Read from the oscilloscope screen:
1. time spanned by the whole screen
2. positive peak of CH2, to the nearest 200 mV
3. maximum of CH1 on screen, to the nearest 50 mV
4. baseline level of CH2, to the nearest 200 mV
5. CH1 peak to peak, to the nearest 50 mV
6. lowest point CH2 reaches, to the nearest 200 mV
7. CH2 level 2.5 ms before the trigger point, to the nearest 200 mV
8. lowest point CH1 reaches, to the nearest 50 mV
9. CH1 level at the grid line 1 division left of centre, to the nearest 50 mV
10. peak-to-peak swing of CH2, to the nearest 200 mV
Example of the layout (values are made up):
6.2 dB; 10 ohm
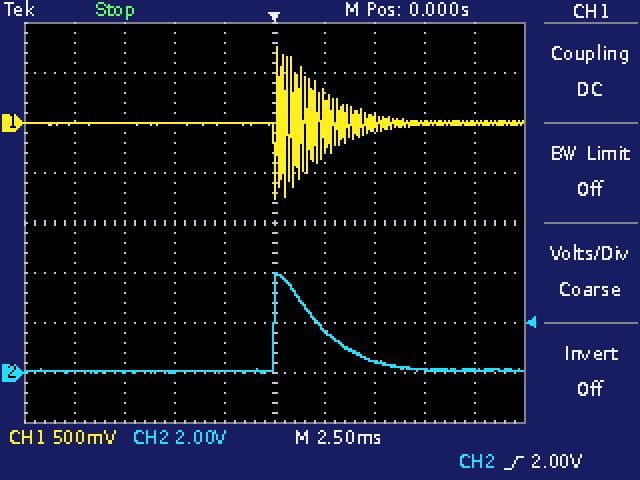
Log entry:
25 ms; 4.0 V; 750 mV; 0.0 V; 1.50 V; 0.0 V; 0.0 V; -750 mV; 0 mV; 4.0 V
